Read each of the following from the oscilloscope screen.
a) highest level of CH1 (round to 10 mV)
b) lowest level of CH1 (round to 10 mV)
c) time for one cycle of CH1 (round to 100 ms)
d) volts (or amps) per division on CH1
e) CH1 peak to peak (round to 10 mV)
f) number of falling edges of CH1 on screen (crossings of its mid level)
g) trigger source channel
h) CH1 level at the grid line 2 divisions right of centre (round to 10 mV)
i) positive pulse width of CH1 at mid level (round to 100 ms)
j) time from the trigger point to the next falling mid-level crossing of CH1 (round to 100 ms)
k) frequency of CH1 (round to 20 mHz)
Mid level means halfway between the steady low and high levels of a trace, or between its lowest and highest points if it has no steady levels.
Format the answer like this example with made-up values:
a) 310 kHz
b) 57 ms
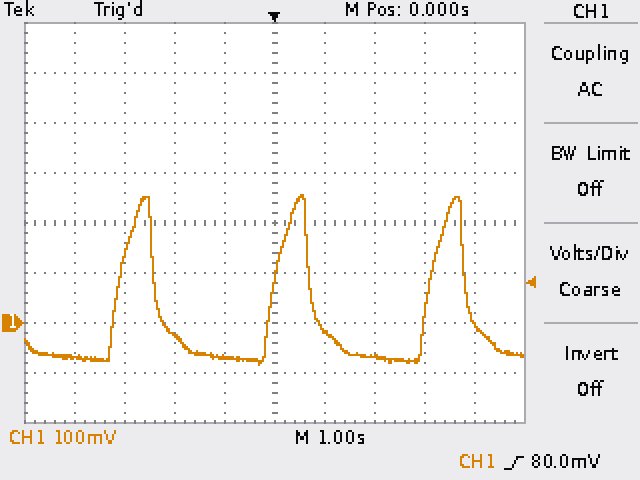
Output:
a) 260 mV
b) -80 mV
c) 3.1 s
d) 100 mV
e) 340 mV
f) 3
g) CH1
h) -70 mV
i) 700 ms
j) 700 ms
k) 320 mHz
